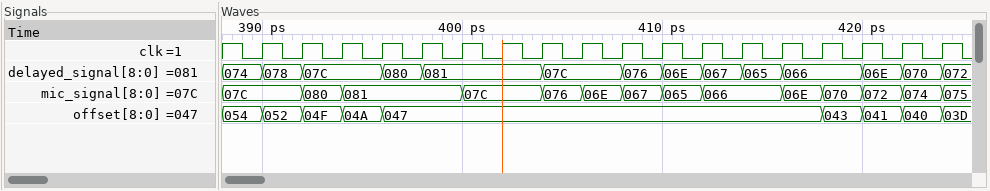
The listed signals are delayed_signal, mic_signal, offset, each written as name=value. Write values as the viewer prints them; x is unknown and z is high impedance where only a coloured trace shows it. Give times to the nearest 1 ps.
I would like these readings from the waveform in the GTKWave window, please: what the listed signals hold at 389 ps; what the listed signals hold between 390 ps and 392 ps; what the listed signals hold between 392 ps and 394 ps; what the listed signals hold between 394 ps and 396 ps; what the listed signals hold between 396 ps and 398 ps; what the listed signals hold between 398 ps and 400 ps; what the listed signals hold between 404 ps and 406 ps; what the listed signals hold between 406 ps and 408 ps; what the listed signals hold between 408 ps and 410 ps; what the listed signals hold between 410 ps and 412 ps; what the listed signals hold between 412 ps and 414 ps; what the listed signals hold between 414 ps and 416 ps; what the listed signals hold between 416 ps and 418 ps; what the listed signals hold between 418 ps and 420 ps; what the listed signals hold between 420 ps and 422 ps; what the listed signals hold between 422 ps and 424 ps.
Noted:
delayed_signal=074, mic_signal=07C, offset=054
delayed_signal=078, mic_signal=07C, offset=052
delayed_signal=07C, mic_signal=080, offset=04F
delayed_signal=07C, mic_signal=081, offset=04A
delayed_signal=080, mic_signal=081, offset=047
delayed_signal=081, mic_signal=081, offset=047
delayed_signal=07C, mic_signal=076, offset=047
delayed_signal=07C, mic_signal=06E, offset=047
delayed_signal=076, mic_signal=067, offset=047
delayed_signal=06E, mic_signal=065, offset=047
delayed_signal=067, mic_signal=066, offset=047
delayed_signal=065, mic_signal=066, offset=047
delayed_signal=066, mic_signal=06E, offset=047
delayed_signal=066, mic_signal=070, offset=043
delayed_signal=06E, mic_signal=072, offset=041
delayed_signal=070, mic_signal=074, offset=040
